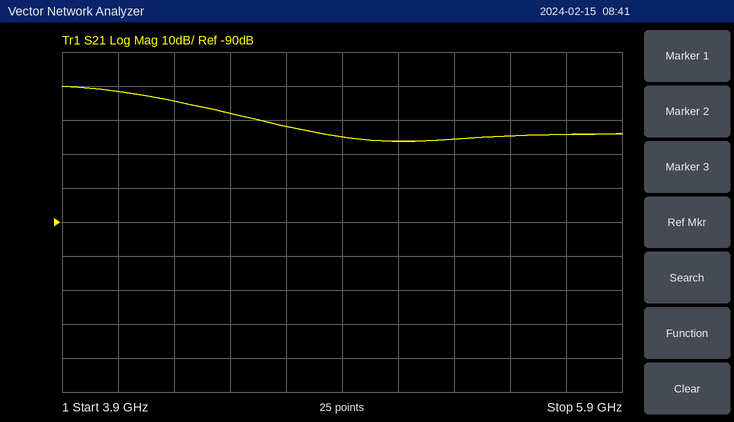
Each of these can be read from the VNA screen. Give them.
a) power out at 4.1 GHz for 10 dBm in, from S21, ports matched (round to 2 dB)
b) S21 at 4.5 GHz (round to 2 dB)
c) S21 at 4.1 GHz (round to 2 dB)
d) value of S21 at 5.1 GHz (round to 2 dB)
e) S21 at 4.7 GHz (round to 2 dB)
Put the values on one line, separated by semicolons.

-42 dBm; -58 dB; -52 dB; -66 dB; -62 dB
